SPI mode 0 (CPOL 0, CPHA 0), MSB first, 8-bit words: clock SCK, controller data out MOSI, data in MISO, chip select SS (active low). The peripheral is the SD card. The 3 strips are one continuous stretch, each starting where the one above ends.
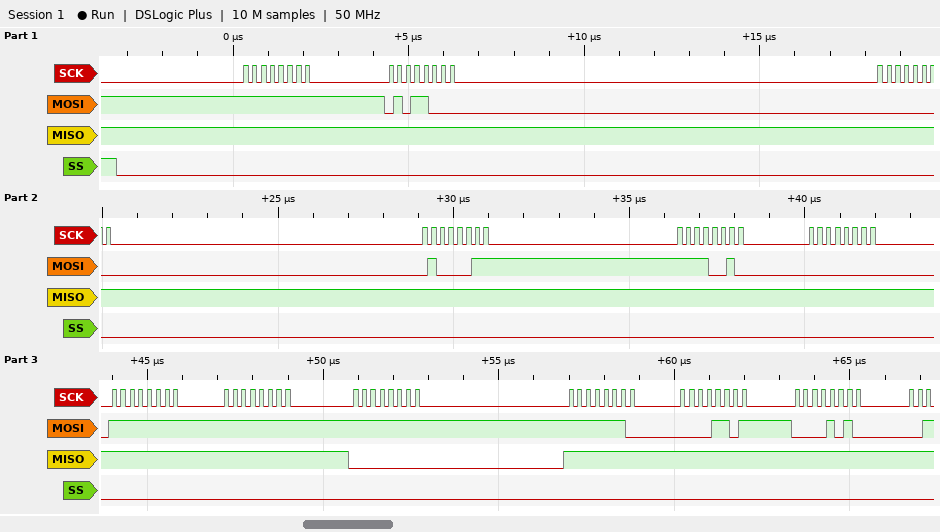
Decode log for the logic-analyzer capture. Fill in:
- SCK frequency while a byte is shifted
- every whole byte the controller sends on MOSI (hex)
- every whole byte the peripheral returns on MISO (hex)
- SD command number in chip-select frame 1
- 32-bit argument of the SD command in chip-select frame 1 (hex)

4 MHz
FF 58 00 43 F2 00 FF FF FF FE 0D 0A
FF FF FF FF FF FF FF FF 00 FF FF FF
CMD24
0x0043F200
